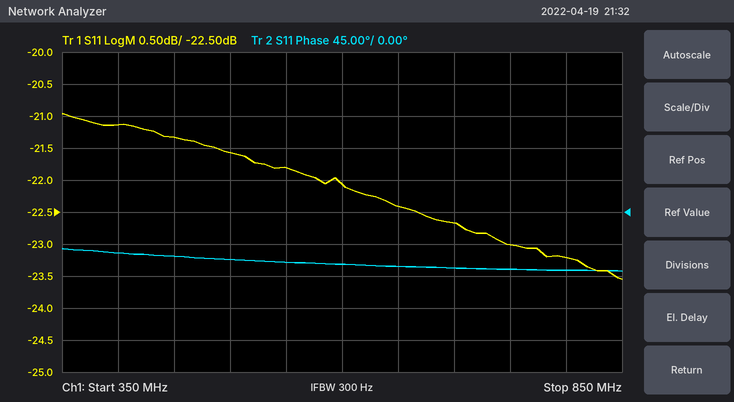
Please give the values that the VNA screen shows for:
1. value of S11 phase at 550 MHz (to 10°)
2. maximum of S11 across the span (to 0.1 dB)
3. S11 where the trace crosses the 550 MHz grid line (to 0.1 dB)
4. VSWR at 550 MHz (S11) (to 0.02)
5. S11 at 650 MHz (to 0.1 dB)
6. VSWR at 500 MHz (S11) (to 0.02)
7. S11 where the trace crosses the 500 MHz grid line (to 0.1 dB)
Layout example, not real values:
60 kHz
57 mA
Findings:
-70°
-21.0 dB
-21.8 dB
1.18
-22.4 dB
1.18
-21.6 dB
